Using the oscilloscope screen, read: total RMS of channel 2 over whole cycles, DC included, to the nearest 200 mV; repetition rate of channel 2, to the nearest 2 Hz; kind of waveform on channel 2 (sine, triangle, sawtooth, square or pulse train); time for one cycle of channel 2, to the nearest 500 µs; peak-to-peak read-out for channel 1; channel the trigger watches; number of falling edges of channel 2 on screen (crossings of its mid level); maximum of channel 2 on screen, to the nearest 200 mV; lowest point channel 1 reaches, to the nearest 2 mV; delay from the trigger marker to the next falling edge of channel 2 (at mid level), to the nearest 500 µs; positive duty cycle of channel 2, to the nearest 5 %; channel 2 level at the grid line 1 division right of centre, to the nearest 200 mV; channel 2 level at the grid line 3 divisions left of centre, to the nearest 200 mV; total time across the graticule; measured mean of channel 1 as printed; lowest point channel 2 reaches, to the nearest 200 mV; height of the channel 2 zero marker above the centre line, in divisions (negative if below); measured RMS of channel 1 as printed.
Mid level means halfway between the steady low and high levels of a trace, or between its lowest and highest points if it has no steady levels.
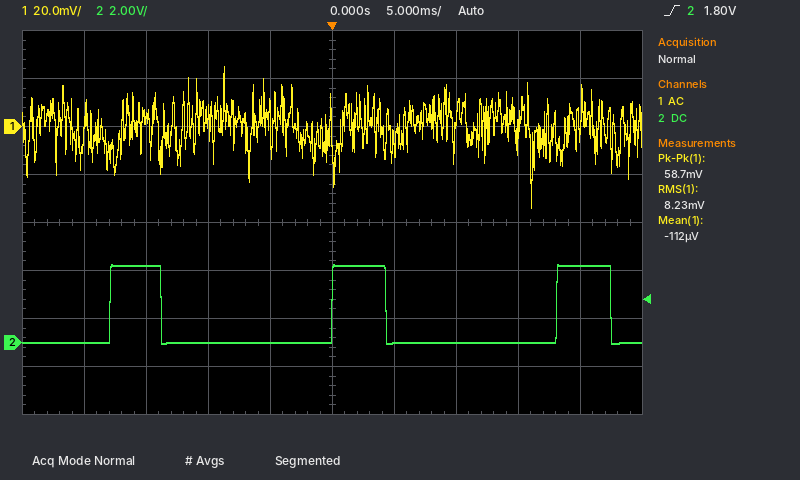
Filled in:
1.6 V
56 Hz
pulse train
18.0 ms
58.7 mV
channel 2
3
3.2 V
-34 mV
4.5 ms
25 %
0.0 V
3.2 V
50 ms
-112 µV
0.0 V
-2.5 div
8.23 mV
